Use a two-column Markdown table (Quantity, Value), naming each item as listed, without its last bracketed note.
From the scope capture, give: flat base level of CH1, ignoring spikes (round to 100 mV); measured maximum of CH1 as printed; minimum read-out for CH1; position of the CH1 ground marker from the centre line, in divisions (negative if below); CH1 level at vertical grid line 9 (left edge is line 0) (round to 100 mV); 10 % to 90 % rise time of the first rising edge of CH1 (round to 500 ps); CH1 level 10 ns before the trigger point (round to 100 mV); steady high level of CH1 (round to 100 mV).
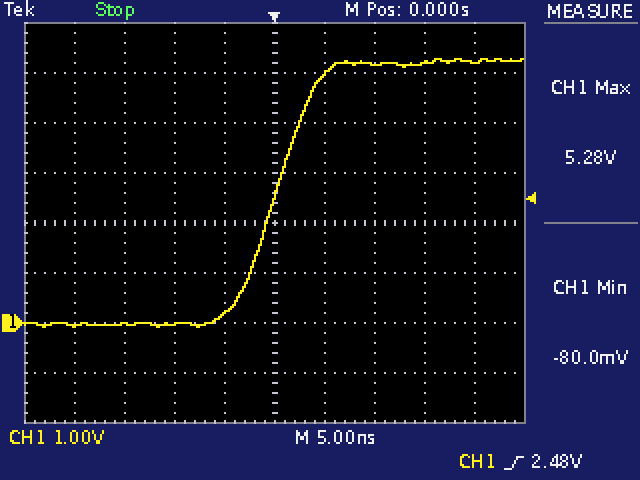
| Quantity | Value |
|---|---|
| flat base level of CH1, ignoring spikes | 0.0 V |
| measured maximum of CH1 as printed | 5.28 V |
| minimum read-out for CH1 | -80.0 mV |
| position of the CH1 ground marker from the centre line, in divisions | -2.0 div |
| CH1 level at vertical grid line 9 (left edge is line 0) | 5.2 V |
| 10 % to 90 % rise time of the first rising edge of CH1 | 7.5 ns |
| CH1 level 10 ns before the trigger point | 0.0 V |
| steady high level of CH1 | 5.2 V |
